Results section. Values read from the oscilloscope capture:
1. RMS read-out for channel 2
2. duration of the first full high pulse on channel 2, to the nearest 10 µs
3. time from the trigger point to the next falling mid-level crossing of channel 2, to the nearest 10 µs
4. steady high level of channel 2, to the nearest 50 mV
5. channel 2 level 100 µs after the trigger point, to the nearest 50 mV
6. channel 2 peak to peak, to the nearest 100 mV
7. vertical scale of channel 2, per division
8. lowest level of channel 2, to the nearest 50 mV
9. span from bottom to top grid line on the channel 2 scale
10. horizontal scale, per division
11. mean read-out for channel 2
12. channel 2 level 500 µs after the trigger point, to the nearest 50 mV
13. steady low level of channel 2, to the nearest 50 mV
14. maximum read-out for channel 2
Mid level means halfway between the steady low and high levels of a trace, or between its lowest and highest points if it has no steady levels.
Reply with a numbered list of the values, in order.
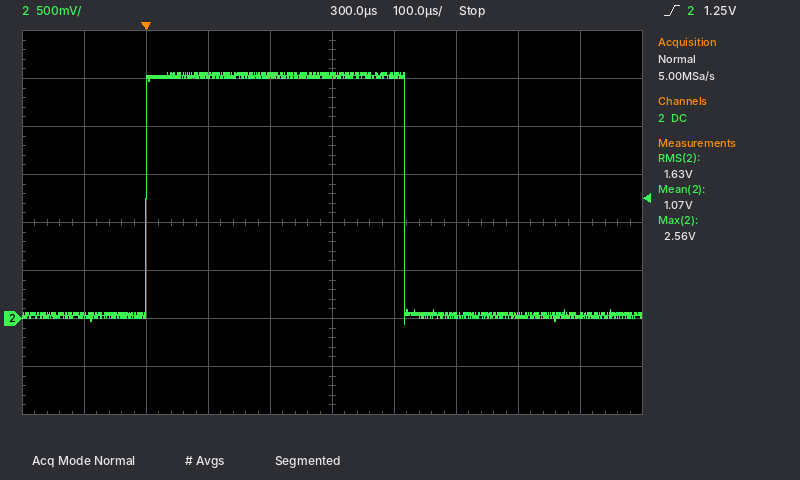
1. 1.63 V
2. 420 µs
3. 420 µs
4. 2.55 V
5. 2.55 V
6. 2.60 V
7. 500 mV
8. -50 mV
9. 4 V
10. 100 µs
11. 1.07 V
12. 50 mV
13. 50 mV
14. 2.56 V
